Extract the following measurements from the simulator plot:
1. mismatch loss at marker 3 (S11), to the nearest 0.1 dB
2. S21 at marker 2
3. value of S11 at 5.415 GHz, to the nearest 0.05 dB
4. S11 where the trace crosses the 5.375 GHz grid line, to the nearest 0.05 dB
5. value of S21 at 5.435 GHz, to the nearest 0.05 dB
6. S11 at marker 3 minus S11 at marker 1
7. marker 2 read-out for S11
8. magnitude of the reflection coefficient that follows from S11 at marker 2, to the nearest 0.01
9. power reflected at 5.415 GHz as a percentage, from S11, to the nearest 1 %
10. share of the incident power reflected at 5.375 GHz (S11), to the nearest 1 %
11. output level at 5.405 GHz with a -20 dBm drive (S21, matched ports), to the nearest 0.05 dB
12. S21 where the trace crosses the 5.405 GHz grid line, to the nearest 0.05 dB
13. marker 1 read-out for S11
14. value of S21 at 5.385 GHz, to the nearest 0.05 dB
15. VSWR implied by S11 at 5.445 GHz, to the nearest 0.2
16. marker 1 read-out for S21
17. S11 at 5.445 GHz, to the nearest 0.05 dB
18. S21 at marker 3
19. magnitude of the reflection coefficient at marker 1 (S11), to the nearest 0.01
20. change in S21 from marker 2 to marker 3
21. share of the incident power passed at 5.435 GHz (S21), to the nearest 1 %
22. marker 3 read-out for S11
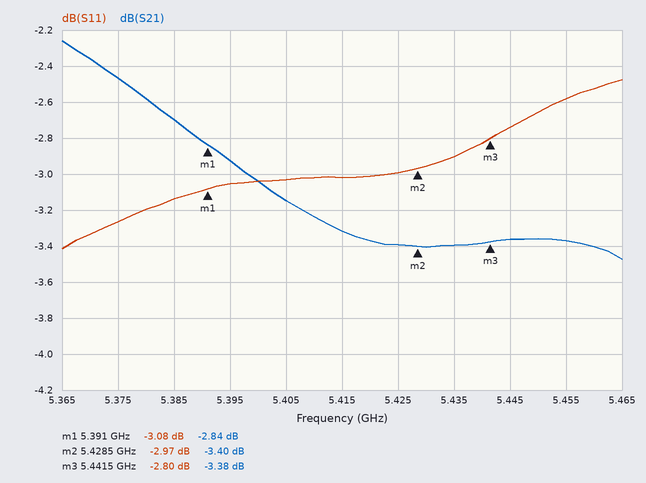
3.2 dB
-3.40 dB
-3.00 dB
-3.25 dB
-3.40 dB
0.28 dB
-2.97 dB
0.71
50 %
47 %
-23.15 dBm
-3.15 dB
-3.08 dB
-2.70 dB
6.4
-2.84 dB
-2.75 dB
-3.38 dB
0.70
0.02 dB
46 %
-2.80 dB
